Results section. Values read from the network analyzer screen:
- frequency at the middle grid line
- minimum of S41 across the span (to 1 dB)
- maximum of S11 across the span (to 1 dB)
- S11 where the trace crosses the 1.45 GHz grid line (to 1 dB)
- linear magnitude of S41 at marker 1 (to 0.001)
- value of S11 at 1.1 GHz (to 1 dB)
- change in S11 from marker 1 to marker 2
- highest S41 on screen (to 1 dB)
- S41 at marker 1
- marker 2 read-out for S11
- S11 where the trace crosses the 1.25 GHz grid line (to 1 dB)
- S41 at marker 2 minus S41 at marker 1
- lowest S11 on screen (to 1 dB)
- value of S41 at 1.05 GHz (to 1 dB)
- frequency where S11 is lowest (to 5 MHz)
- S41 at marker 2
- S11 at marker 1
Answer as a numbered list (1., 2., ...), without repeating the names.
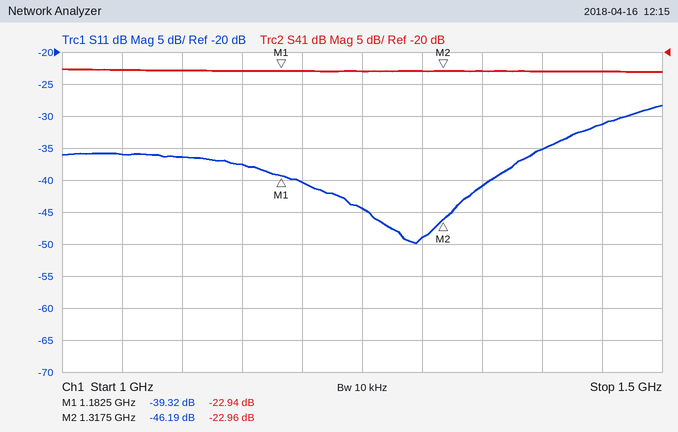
1. 1.25 GHz
2. -23 dB
3. -28 dB
4. -31 dB
5. 0.071
6. -36 dB
7. -6.87 dB
8. -23 dB
9. -22.94 dB
10. -46.19 dB
11. -44 dB
12. -0.02 dB
13. -50 dB
14. -23 dB
15. 1.295 GHz
16. -22.96 dB
17. -39.32 dB
